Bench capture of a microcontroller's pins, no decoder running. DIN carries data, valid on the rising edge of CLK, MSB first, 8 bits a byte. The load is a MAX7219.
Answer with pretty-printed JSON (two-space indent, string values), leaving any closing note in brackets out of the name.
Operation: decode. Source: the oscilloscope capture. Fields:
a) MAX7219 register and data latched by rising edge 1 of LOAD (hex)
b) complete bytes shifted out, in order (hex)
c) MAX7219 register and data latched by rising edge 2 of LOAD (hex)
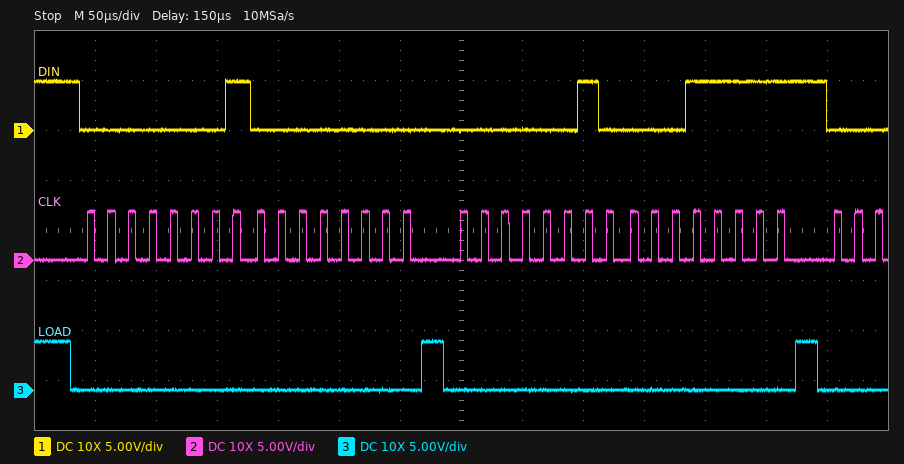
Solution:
{
  "MAX7219 register and data latched by rising edge 1 of LOAD": "register 0x1, data 0x00",
  "complete bytes shifted out, in order": "01 00 02 1F",
  "MAX7219 register and data latched by rising edge 2 of LOAD": "register 0x2, data 0x1F"
}
